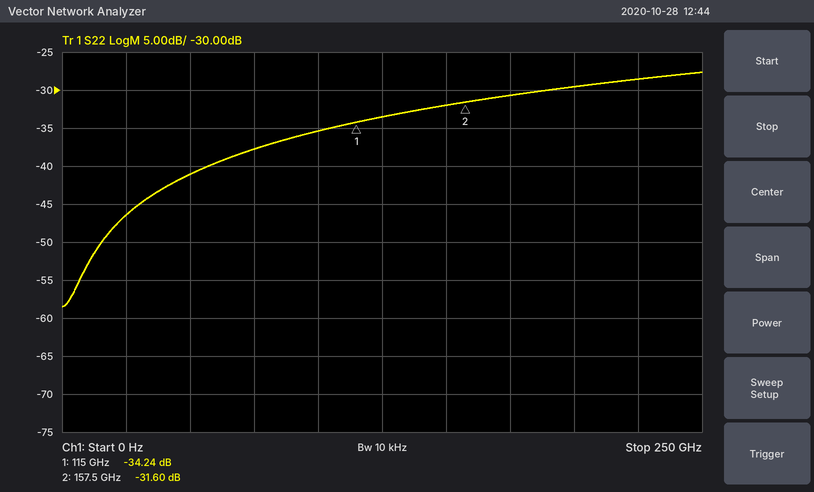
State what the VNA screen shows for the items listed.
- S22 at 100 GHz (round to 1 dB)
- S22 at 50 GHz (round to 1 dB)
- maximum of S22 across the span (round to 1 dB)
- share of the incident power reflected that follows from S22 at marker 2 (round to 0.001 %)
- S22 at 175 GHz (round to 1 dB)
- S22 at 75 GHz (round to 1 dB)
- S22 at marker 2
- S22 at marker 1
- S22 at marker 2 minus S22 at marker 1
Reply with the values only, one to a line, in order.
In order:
-35 dB
-41 dB
-28 dB
0.069 %
-31 dB
-38 dB
-31.60 dB
-34.24 dB
2.64 dB
